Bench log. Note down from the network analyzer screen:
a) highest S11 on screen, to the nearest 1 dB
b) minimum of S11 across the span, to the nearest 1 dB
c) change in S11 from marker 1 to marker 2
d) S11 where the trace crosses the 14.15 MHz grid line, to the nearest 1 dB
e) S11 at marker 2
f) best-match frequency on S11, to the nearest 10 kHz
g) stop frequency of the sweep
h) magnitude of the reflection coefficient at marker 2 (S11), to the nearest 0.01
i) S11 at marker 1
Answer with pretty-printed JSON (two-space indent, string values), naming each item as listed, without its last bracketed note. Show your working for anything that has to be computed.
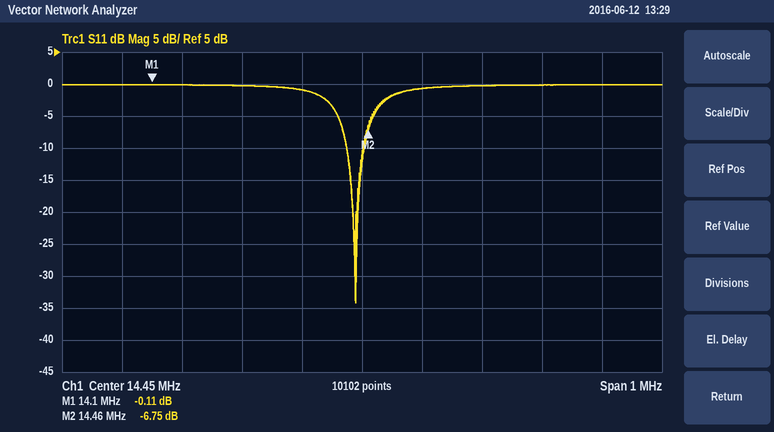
{
  "highest S11 on screen, to the nearest 1 dB": "0 dB",
  "minimum of S11 across the span, to the nearest 1 dB": "-34 dB",
  "change in S11 from marker 1 to marker 2": "-6.75 − (-0.11) = -6.64 dB",
  "S11 where the trace crosses the 14.15 MHz grid line, to the nearest 1 dB": "0 dB",
  "S11 at marker 2": "-6.75 dB",
  "best-match frequency on S11, to the nearest 10 kHz": "14.44 MHz",
  "stop frequency of the sweep": "14.95 MHz",
  "magnitude of the reflection coefficient at marker 2 (S11), to the nearest 0.01": "10^(-6.75/20) ≈ 0.46",
  "S11 at marker 1": "-0.11 dB"
}
